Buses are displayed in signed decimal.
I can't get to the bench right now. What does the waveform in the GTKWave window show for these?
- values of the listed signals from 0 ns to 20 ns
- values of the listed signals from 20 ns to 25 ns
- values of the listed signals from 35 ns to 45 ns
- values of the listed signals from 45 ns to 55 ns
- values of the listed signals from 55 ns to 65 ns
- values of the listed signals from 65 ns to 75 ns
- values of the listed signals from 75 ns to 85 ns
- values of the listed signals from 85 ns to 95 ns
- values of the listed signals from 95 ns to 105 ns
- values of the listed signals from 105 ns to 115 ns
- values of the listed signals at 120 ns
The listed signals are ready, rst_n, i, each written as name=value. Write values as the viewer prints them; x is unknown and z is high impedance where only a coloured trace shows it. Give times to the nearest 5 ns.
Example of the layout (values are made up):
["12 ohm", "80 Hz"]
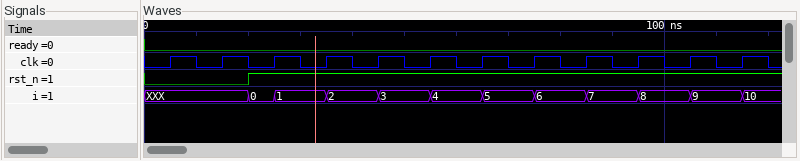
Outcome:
["ready=0, rst_n=0, i=XXX", "ready=0, rst_n=1, i=0", "ready=0, rst_n=1, i=2", "ready=0, rst_n=1, i=3", "ready=0, rst_n=1, i=4", "ready=0, rst_n=1, i=5", "ready=0, rst_n=1, i=6", "ready=0, rst_n=1, i=7", "ready=0, rst_n=1, i=8", "ready=0, rst_n=1, i=9", "ready=0, rst_n=1, i=10"]
